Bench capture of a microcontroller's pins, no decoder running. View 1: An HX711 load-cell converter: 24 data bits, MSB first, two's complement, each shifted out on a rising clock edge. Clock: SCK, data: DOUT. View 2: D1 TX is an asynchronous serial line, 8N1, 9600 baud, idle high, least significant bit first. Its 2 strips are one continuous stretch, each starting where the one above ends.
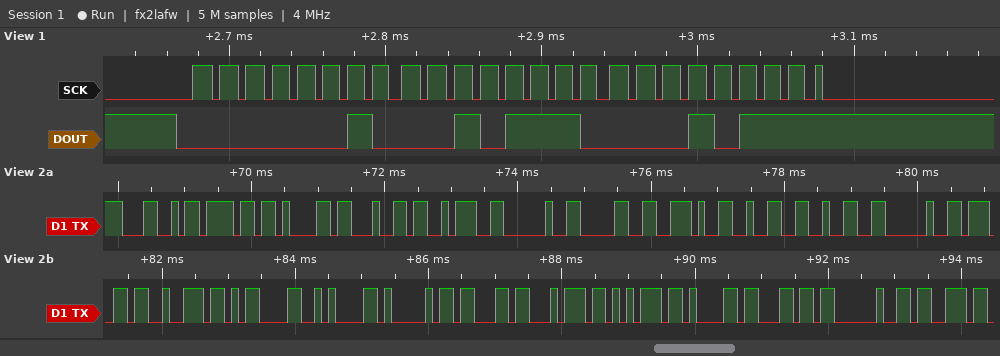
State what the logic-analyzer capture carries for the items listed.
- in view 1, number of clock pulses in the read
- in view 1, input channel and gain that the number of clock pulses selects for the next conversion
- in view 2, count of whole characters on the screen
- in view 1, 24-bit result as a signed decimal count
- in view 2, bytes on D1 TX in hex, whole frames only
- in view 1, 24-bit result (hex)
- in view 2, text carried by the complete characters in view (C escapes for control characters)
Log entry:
25
channel A, gain 128
23
142871
4C 6F 61 64 3A 20 30 2E 32 32 20 67 72 0D 0A 41 63 74 75 61 6C 20 73
0x022E17
"Load: 0.22 gr\r\nActual s"
